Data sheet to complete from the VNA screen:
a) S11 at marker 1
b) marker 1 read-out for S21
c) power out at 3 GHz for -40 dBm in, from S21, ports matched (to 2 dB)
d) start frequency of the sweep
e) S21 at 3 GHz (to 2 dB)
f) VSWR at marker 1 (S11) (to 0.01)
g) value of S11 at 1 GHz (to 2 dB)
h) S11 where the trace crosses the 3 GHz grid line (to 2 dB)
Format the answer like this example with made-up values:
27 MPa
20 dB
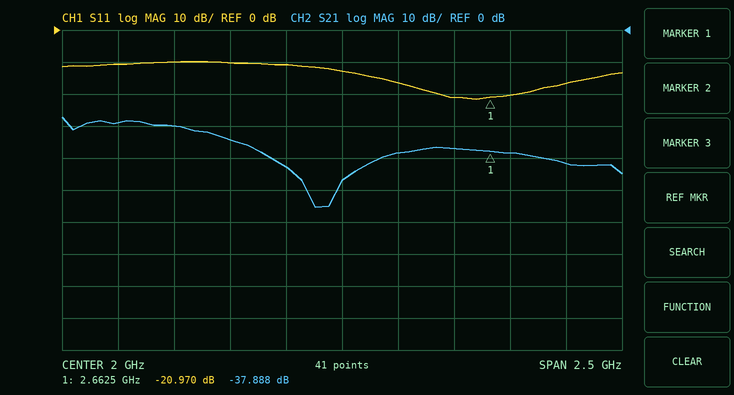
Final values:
-20.970 dB
-37.888 dB
-82 dBm
750 MHz
-42 dB
1.20
-10 dB
-16 dB
